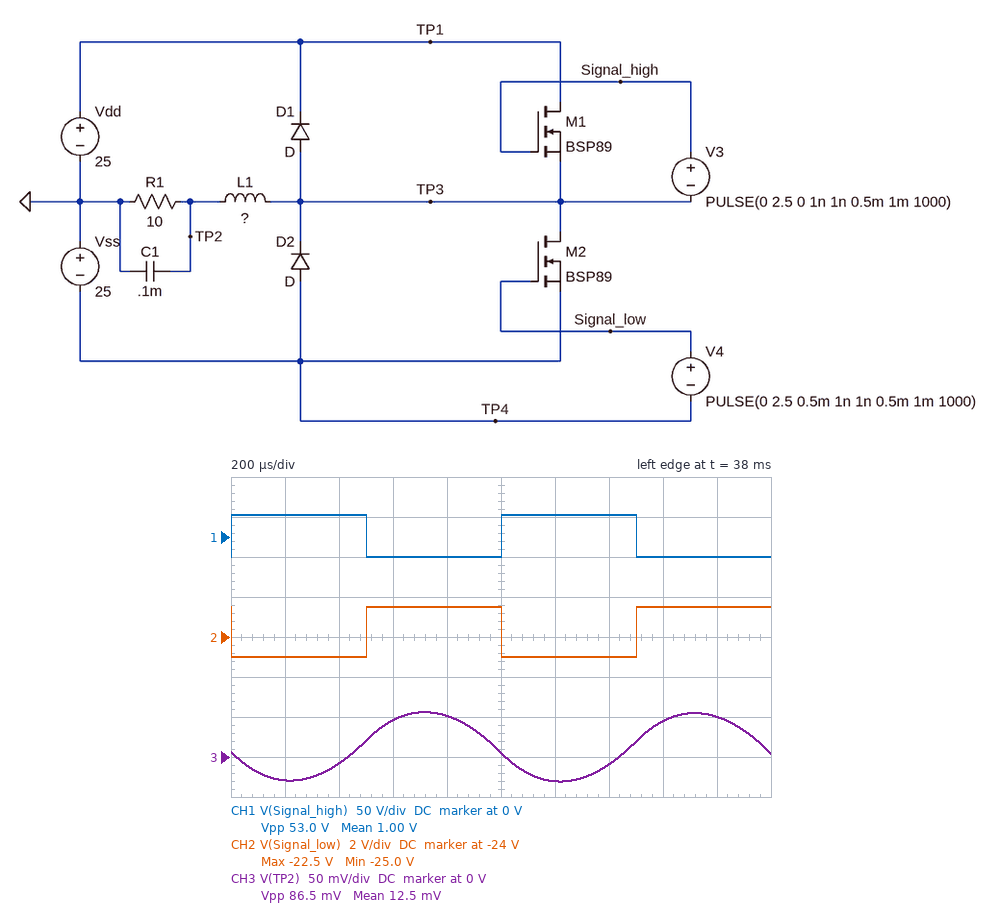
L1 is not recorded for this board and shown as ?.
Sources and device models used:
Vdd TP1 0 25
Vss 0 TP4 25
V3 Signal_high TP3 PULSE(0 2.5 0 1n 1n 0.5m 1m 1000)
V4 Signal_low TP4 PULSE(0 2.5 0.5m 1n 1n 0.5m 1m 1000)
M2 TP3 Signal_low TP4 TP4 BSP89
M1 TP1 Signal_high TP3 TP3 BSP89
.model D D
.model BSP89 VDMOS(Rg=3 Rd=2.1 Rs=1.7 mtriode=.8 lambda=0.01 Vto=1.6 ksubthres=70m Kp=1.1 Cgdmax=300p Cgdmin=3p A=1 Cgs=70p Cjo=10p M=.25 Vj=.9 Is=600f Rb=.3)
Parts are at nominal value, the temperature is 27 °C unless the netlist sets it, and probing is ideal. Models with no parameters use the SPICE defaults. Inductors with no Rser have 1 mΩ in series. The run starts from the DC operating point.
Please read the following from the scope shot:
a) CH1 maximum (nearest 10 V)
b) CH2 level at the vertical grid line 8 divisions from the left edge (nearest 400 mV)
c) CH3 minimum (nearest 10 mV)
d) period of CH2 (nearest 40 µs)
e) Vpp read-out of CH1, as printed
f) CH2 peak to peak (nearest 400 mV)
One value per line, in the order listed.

30 V
-22.4 V
-30 mV
1.00 ms
53.0 V
2.4 V
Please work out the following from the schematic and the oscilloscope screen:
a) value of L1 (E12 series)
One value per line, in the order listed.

180 mH
